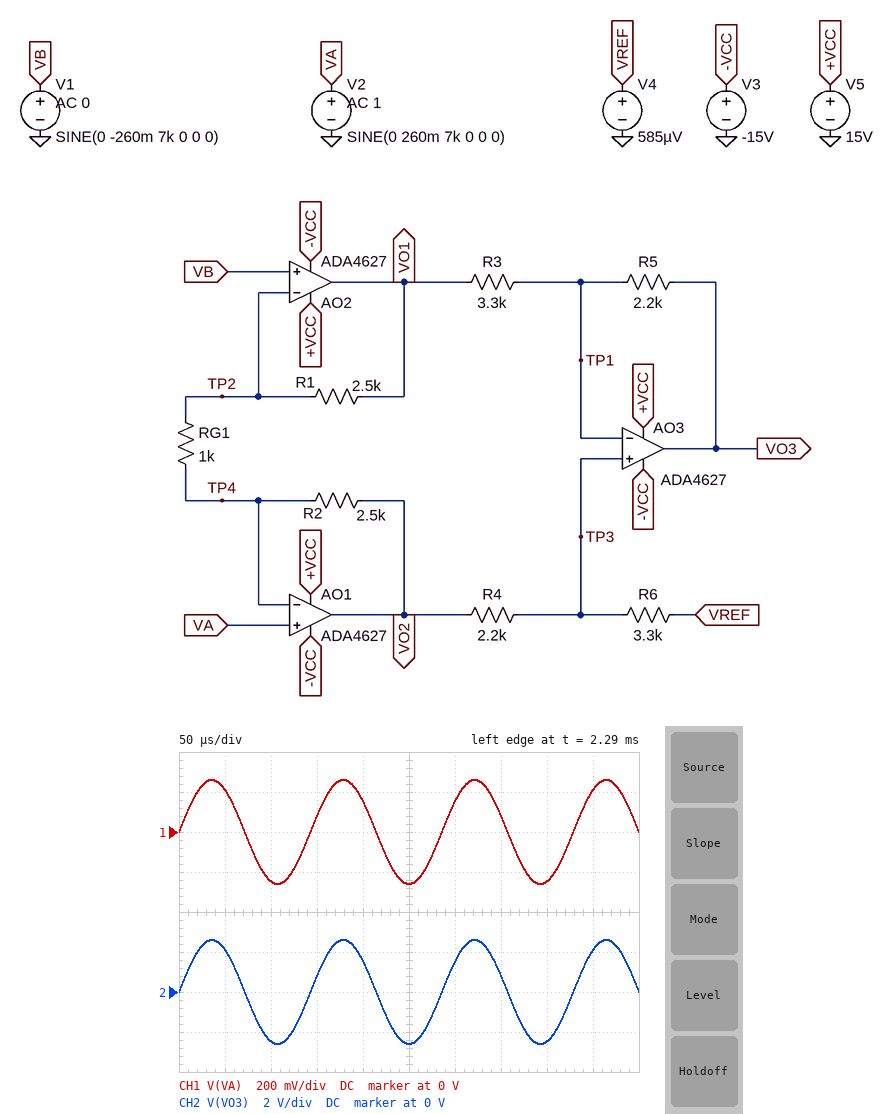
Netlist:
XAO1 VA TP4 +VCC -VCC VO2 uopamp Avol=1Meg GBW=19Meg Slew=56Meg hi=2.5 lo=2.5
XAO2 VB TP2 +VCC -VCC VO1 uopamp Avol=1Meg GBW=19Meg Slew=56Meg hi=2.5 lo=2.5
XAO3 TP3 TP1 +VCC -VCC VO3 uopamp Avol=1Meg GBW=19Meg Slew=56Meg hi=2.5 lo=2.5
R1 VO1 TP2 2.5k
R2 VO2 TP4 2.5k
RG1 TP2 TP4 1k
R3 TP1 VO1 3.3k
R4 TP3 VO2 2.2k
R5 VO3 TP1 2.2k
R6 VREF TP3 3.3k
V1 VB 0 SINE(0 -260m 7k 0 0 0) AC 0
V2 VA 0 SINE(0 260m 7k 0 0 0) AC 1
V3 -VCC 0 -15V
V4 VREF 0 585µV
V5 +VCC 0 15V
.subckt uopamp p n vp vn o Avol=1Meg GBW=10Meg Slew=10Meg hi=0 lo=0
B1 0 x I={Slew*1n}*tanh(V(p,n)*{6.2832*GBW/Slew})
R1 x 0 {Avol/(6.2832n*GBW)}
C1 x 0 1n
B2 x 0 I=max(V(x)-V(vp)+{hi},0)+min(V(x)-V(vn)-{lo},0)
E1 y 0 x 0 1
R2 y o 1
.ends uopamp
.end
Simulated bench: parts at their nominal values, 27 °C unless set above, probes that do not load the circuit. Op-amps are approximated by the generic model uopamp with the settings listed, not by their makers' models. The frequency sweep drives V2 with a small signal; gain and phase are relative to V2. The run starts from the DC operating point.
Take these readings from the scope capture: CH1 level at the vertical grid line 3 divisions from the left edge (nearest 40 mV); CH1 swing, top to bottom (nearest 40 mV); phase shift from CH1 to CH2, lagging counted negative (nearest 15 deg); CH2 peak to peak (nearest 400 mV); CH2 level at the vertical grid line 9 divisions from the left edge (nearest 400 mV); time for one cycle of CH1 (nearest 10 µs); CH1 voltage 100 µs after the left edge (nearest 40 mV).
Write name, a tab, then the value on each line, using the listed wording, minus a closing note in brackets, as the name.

CH1 level at the vertical grid line 3 divisions from the left edge	80 mV
CH1 swing, top to bottom	520 mV
phase shift from CH1 to CH2, lagging counted negative	0 deg
CH2 peak to peak	5.2 V
CH2 level at the vertical grid line 9 divisions from the left edge	2.0 V
time for one cycle of CH1	140 µs
CH1 voltage 100 µs after the left edge	-240 mV
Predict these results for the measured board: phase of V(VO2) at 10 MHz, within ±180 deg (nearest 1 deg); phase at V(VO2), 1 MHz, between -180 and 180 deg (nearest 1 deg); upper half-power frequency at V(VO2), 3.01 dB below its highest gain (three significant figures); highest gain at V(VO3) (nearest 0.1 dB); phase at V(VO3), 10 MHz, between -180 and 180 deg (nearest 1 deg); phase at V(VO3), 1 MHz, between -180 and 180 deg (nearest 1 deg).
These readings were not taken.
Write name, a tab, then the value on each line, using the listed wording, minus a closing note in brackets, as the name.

phase of V(VO2) at 10 MHz, within ±180 deg	-58 deg
phase at V(VO2), 1 MHz, between -180 and 180 deg	-15 deg
upper half-power frequency at V(VO2), 3.01 dB below its highest gain	3.34 MHz
highest gain at V(VO3)	14.3 dB
phase at V(VO3), 10 MHz, between -180 and 180 deg	-110 deg
phase at V(VO3), 1 MHz, between -180 and 180 deg	-22 deg
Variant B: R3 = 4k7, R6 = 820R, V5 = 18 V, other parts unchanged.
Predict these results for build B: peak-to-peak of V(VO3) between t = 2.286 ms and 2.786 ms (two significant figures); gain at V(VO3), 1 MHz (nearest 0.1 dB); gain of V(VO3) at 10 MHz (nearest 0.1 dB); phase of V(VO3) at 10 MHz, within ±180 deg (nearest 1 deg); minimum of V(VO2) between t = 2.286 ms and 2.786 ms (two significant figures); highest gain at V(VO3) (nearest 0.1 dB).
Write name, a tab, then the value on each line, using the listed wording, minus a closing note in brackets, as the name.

peak-to-peak of V(VO3) between t = 2.286 ms and 2.786 ms	2.7 V
gain at V(VO3), 1 MHz	7.7 dB
gain of V(VO3) at 10 MHz	-4.4 dB
phase of V(VO3) at 10 MHz, within ±180 deg	-112 deg
minimum of V(VO2) between t = 2.286 ms and 2.786 ms	-1.6 V
highest gain at V(VO3)	8.2 dB
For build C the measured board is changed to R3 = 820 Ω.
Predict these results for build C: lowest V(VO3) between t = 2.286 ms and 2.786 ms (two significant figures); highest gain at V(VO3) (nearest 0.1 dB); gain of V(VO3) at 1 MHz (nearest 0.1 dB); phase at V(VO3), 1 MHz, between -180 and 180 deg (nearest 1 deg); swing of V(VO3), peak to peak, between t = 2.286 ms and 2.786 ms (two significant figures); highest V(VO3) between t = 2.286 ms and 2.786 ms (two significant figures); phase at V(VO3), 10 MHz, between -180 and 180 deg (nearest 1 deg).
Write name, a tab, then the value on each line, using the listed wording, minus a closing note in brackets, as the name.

lowest V(VO3) between t = 2.286 ms and 2.786 ms	-7.6 V
highest gain at V(VO3)	23.2 dB
gain of V(VO3) at 1 MHz	22.6 dB
phase at V(VO3), 1 MHz, between -180 and 180 deg	-29 deg
swing of V(VO3), peak to peak, between t = 2.286 ms and 2.786 ms	15 V
highest V(VO3) between t = 2.286 ms and 2.786 ms	7.6 V
phase at V(VO3), 10 MHz, between -180 and 180 deg	-137 deg
